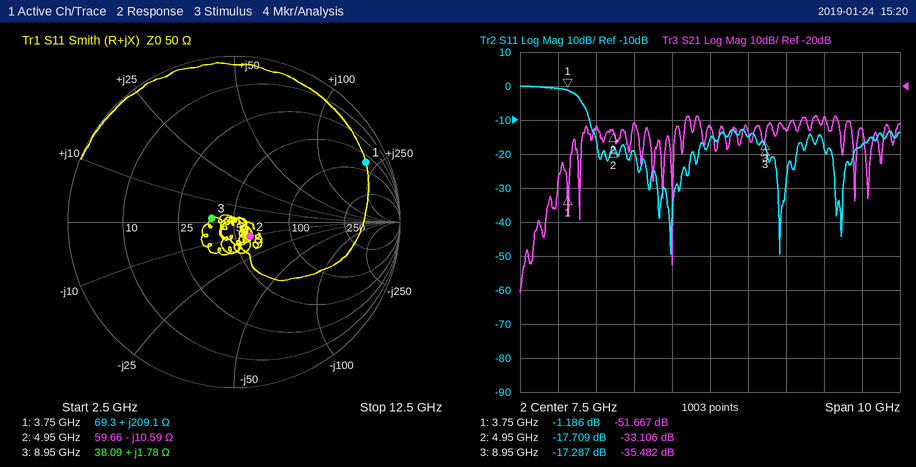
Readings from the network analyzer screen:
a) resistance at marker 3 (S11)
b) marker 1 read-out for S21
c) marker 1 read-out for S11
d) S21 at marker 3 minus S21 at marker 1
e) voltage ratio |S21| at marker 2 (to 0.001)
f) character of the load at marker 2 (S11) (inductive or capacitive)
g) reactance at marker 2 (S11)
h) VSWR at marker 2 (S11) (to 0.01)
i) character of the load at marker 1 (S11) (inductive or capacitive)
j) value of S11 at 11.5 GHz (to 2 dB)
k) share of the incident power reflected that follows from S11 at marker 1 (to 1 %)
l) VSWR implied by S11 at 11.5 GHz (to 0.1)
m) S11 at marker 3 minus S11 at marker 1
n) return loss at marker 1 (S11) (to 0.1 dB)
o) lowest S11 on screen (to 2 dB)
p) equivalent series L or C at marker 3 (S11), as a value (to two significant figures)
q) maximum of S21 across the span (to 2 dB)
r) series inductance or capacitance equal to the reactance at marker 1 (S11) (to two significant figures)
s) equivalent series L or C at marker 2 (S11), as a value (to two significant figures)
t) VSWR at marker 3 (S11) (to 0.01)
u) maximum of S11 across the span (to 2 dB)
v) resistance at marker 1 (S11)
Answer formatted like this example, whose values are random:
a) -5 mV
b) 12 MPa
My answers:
a) 38.09 Ω
b) -51.667 dB
c) -1.186 dB
d) 16.185 dB
e) 0.022
f) capacitive
g) -10.59 Ω
h) 1.30
i) inductive
j) -18 dB
k) 76 %
l) 1.3
m) -16.101 dB
n) 1.2 dB
o) -50 dB
p) 32 pH
q) -28 dB
r) 8.9 nH
s) 3.0 pF
t) 1.32
u) 0 dB
v) 69.3 Ω
